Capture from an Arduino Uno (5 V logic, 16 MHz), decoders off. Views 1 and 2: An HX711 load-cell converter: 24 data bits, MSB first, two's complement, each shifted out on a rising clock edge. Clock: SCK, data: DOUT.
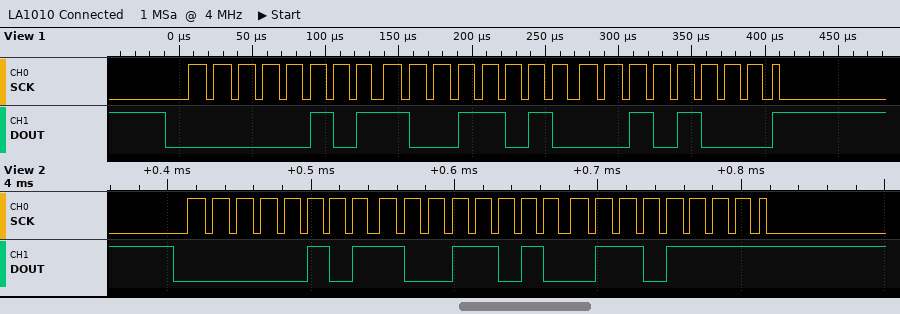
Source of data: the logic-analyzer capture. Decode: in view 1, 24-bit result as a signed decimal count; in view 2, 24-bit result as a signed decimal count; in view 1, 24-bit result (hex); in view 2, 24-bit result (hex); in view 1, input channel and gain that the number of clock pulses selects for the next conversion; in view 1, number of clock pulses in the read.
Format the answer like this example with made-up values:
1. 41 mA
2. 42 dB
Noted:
1. 367144
2. 367215
3. 0x059A28
4. 0x059A6F
5. channel A, gain 128
6. 25
